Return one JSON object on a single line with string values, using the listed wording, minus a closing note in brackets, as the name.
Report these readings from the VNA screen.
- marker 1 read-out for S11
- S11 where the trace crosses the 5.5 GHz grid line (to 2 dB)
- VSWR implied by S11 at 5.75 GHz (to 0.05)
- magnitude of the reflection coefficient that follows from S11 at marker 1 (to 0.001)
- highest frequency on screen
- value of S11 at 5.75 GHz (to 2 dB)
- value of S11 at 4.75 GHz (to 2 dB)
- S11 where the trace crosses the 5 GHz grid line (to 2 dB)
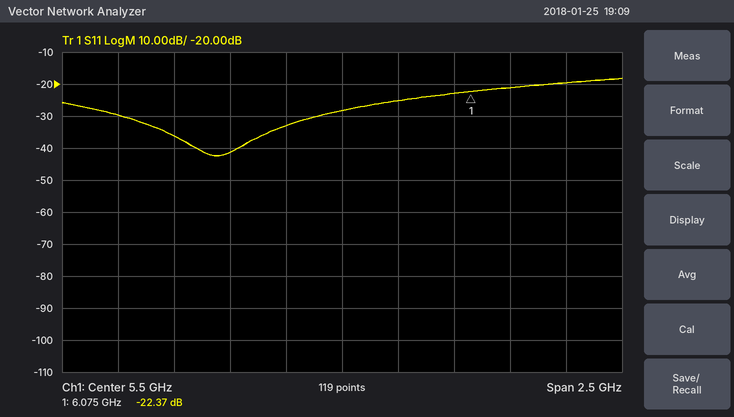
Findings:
{"marker 1 read-out for S11": "-22.37 dB", "S11 where the trace crosses the 5.5 GHz grid line": "-28 dB", "VSWR implied by S11 at 5.75 GHz": "1.10", "magnitude of the reflection coefficient that follows from S11 at marker 1": "0.076", "highest frequency on screen": "6.75 GHz", "value of S11 at 5.75 GHz": "-26 dB", "value of S11 at 4.75 GHz": "-36 dB", "S11 where the trace crosses the 5 GHz grid line": "-42 dB"}
